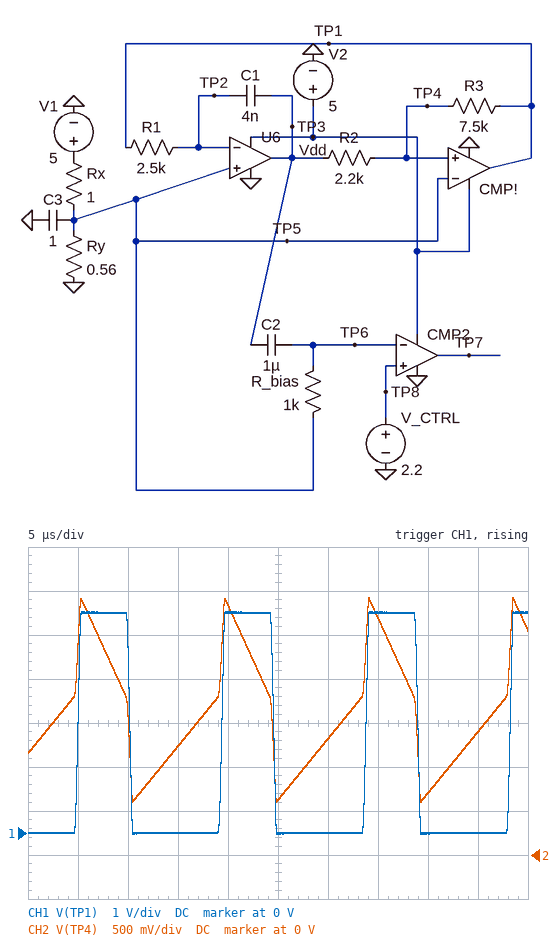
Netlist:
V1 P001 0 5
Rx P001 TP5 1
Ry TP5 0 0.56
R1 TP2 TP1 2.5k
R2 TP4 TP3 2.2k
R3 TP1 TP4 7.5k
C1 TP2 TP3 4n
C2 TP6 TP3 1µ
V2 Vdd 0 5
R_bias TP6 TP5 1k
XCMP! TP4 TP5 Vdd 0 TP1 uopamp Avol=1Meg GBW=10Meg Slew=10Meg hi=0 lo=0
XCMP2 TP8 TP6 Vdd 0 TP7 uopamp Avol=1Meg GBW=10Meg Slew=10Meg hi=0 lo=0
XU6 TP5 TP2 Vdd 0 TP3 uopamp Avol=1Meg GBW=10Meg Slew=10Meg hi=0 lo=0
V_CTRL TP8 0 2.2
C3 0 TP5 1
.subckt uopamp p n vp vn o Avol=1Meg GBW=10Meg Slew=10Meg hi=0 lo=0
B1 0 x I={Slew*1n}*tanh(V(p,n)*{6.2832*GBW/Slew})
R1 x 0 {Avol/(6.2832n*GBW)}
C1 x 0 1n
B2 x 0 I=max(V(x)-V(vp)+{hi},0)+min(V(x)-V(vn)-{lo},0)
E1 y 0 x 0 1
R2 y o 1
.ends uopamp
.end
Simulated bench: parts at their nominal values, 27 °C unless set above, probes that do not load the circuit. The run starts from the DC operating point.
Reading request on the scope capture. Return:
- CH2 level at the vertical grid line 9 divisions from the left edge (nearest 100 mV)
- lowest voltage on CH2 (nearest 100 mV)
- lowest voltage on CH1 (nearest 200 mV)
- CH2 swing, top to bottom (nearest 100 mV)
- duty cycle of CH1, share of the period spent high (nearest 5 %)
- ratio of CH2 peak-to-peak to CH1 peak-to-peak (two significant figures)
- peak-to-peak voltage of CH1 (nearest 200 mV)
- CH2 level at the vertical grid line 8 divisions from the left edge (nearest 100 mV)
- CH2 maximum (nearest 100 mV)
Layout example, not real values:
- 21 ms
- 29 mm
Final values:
- 1.4 V
- 600 mV
- 0 V
- 2.3 V
- 35 %
- 0.46
- 5.0 V
- 700 mV
- 2.9 V
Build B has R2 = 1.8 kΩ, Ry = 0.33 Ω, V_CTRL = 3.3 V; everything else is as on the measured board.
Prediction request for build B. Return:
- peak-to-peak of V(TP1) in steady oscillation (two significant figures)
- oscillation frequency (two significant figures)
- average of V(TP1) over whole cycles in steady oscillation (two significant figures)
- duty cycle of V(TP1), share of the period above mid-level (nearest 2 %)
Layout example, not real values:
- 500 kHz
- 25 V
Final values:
- 5.0 V
- 67 kHz
- 1.2 V
- 24 %
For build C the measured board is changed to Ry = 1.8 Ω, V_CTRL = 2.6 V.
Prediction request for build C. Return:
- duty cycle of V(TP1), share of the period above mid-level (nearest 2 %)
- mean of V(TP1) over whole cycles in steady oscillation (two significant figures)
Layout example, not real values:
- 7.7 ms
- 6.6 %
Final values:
- 64 %
- 3.2 V
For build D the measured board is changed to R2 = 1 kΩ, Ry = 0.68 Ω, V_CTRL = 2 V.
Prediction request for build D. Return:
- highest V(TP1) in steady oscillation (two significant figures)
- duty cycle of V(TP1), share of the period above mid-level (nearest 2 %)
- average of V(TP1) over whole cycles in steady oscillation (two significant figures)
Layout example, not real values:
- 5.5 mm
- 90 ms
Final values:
- 5.0 V
- 40 %
- 2.0 V
